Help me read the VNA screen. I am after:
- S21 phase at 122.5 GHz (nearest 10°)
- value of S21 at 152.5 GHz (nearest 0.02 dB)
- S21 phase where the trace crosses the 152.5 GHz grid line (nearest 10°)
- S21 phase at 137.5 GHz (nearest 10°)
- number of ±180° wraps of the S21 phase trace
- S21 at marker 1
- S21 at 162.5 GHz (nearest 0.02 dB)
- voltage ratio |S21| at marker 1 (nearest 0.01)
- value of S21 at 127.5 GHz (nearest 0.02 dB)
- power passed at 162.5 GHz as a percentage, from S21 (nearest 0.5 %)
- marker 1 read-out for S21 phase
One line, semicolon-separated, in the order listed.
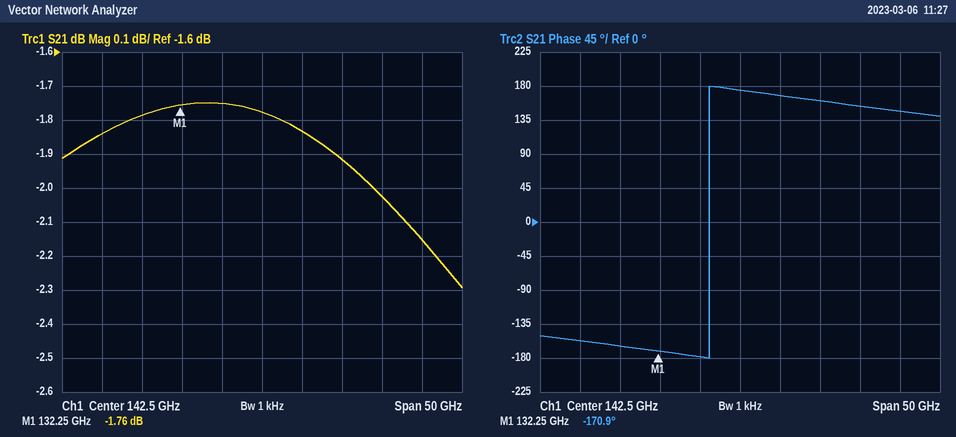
-160°; -1.92 dB; 160°; -180°; 1; -1.76 dB; -2.16 dB; 0.82; -1.78 dB; 61.0 %; -170.9°
